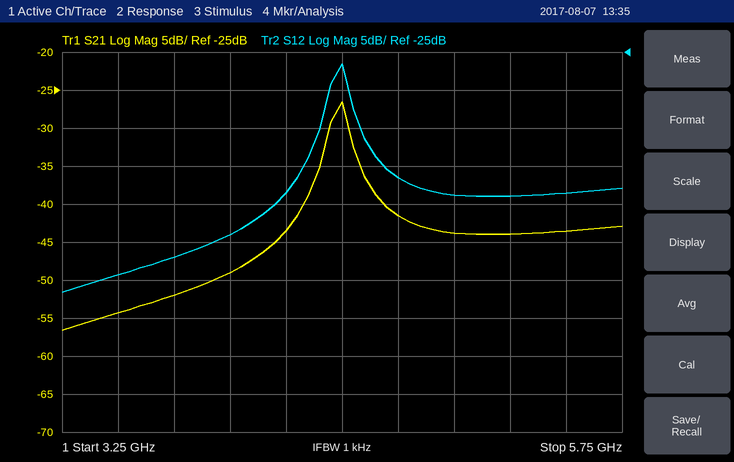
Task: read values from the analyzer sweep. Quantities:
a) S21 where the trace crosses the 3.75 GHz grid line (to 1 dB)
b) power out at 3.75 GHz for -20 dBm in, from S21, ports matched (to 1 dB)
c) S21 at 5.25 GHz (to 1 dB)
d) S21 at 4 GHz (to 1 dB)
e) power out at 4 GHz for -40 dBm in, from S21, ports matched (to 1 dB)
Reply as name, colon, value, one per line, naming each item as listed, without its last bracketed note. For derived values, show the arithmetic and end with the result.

S21 where the trace crosses the 3.75 GHz grid line: -52 dB
power out at 3.75 GHz for -20 dBm in, from S21, ports matched: -20 dBm + (-52 dB) = -72 dBm
S21 at 5.25 GHz: -44 dB
S21 at 4 GHz: -49 dB
power out at 4 GHz for -40 dBm in, from S21, ports matched: -40 dBm + (-49 dB) = -89 dBm
